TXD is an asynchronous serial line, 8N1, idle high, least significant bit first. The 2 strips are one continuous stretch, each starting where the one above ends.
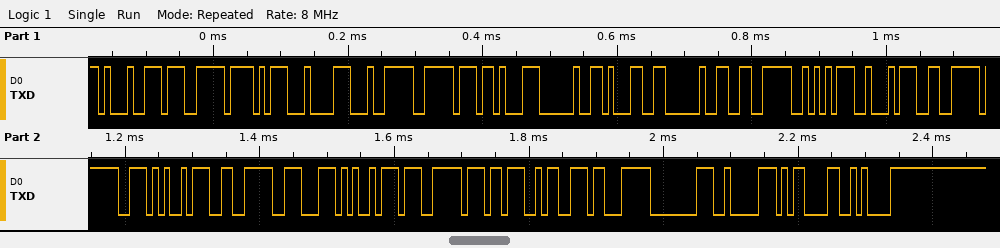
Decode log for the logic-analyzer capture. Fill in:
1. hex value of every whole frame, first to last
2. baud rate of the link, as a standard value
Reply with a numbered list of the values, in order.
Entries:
1. 91 E7 AF 84 E4 BE 8B 20 31 20 E6 AA A2 E6 9F A5 E6 8E A5 E7 B7 9A E3 80 82 0D 0A
2. 115200 baud
